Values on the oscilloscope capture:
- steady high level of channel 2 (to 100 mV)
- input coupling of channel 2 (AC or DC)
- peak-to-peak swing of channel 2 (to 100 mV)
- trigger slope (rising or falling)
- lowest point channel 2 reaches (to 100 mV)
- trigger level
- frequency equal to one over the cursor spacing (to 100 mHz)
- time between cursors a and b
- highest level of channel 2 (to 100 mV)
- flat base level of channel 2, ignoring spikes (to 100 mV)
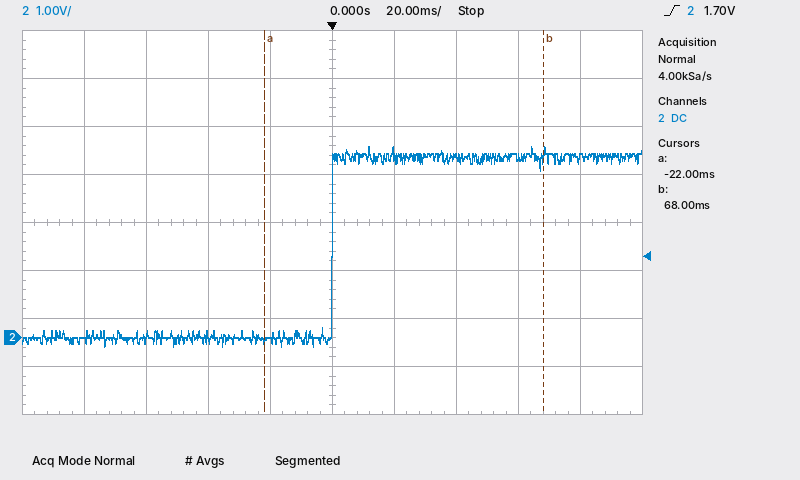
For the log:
3.8 V
DC
4.2 V
rising
-200 mV
1.70 V
11.1 Hz
90 ms
4.0 V
0.0 V
